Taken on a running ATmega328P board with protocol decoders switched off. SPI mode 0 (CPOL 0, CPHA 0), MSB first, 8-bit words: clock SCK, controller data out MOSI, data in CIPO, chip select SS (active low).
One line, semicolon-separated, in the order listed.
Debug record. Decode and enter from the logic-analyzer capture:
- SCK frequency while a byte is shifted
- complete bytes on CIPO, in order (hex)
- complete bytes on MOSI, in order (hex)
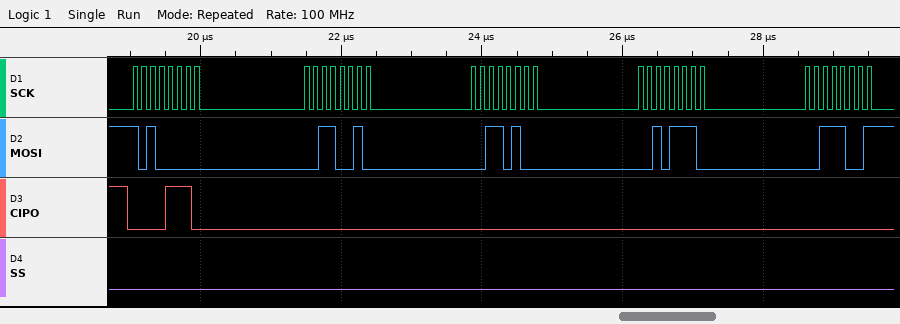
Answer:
8 MHz; 0E 00 00 00 00; A0 32 34 2E 39
